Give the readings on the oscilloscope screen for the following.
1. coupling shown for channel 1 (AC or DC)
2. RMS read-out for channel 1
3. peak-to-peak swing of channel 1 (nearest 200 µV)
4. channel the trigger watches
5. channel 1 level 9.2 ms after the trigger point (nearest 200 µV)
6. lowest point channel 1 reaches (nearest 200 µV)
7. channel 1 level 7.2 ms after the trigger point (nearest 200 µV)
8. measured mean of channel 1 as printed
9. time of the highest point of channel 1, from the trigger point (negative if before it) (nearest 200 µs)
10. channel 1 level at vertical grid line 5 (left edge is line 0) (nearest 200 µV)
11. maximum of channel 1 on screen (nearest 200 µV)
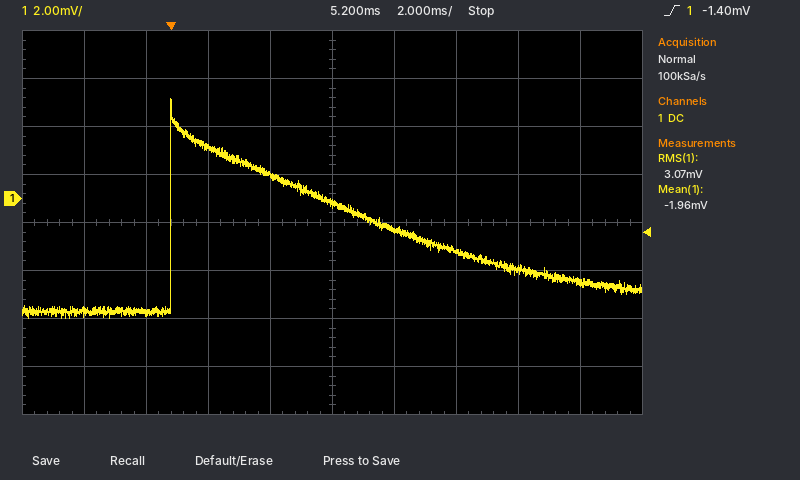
DC
3.07 mV
9.2 mV
channel 1
-2.2 mV
-5.0 mV
-1.2 mV
-1.96 mV
0.0 ms
-200 µV
4.2 mV
